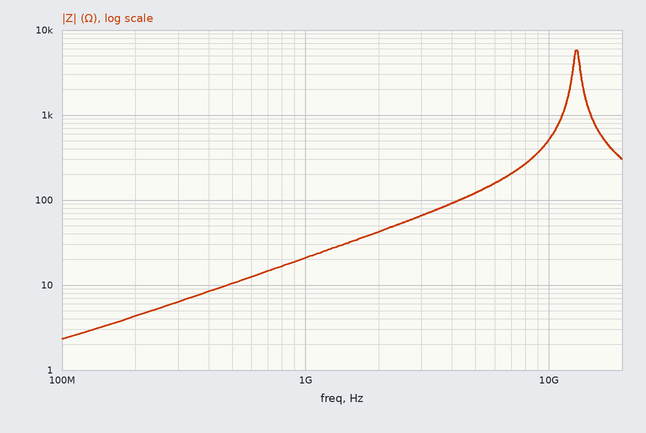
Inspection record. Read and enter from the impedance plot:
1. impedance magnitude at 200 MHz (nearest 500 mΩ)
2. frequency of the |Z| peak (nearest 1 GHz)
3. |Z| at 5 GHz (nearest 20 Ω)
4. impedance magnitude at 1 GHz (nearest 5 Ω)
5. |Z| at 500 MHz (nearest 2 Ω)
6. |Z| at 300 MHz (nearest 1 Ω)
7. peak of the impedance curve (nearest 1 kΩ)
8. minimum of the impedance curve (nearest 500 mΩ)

4.5 Ω
13 GHz
120 Ω
20 Ω
10 Ω
6 Ω
6 kΩ
2.5 Ω
